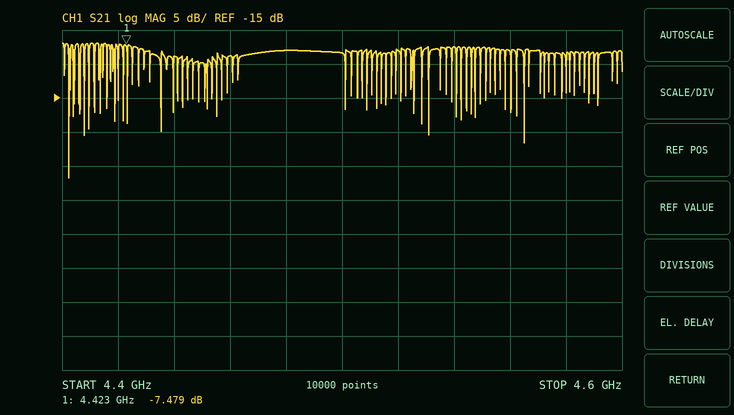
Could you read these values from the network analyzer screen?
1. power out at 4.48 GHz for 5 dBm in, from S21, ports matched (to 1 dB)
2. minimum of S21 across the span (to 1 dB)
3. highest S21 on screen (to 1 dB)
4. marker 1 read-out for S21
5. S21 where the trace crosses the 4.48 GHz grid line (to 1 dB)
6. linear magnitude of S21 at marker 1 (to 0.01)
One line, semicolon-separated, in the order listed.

-3 dBm; -27 dB; -7 dB; -7.479 dB; -8 dB; 0.42
